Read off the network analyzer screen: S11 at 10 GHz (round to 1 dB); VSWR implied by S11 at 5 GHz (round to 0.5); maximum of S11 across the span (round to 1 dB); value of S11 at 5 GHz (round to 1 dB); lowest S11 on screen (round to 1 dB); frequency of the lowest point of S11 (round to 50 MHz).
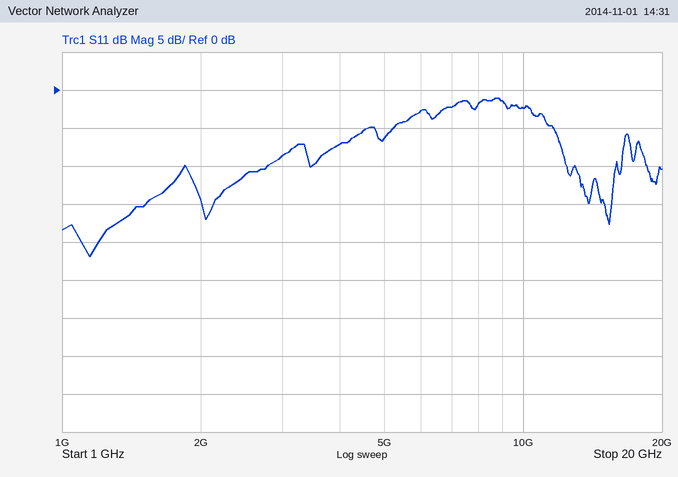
-2 dB
3.0
-1 dB
-6 dB
-22 dB
1.15 GHz
